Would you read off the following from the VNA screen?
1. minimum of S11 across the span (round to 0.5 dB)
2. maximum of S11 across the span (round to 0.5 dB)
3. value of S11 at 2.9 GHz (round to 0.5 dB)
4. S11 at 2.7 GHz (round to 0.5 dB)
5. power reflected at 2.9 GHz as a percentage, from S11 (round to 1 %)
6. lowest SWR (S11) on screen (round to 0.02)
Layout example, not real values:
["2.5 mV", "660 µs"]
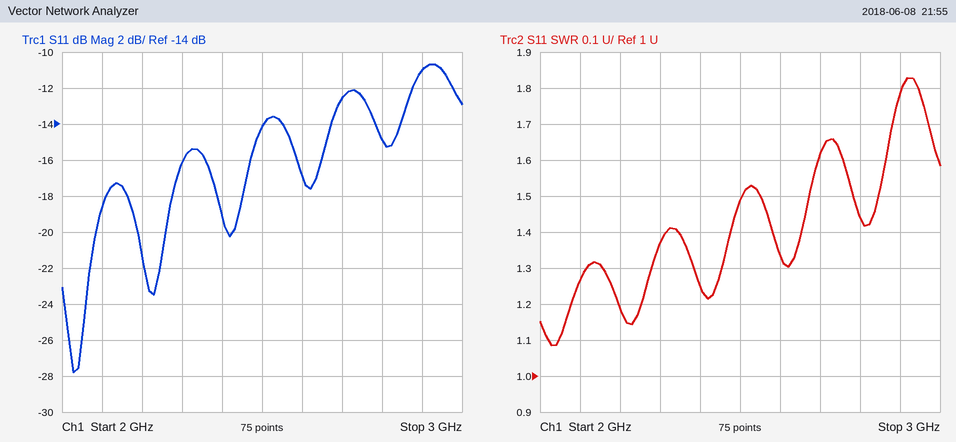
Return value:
["-28.0 dB", "-10.5 dB", "-11.0 dB", "-12.5 dB", "8 %", "1.08"]
